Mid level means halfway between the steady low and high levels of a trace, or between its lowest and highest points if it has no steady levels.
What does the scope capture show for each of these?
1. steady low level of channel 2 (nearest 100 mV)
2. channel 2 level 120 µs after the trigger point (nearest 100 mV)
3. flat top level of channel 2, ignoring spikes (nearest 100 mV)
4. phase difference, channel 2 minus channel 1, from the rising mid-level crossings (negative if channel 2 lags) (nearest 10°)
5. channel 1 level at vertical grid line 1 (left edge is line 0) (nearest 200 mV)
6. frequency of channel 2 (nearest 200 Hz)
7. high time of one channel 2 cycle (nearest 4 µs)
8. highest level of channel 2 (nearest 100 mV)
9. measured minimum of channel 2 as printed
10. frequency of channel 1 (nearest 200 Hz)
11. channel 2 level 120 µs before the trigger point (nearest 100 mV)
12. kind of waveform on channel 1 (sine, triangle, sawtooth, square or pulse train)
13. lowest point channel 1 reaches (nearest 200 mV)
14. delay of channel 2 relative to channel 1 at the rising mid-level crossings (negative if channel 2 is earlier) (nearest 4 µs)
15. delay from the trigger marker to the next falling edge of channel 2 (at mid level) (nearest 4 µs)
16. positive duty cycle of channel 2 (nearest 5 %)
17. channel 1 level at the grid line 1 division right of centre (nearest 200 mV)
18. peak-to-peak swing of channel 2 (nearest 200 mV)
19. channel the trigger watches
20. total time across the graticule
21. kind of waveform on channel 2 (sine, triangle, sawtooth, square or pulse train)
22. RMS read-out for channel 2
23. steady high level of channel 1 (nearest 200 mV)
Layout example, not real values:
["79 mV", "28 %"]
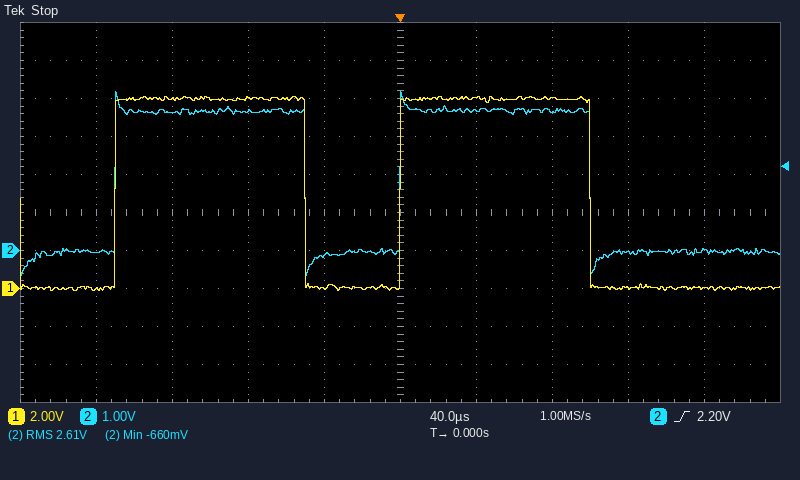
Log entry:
["0.0 V", "-100 mV", "3.7 V", "0°", "0.0 V", "6.6 kHz", "100 µs", "4.2 V", "-660 mV", "6.6 kHz", "3.6 V", "pulse train", "-200 mV", "0 µs", "100 µs", "65 %", "10.0 V", "4.8 V", "channel 2", "400 µs", "pulse train", "2.61 V", "10.0 V"]
